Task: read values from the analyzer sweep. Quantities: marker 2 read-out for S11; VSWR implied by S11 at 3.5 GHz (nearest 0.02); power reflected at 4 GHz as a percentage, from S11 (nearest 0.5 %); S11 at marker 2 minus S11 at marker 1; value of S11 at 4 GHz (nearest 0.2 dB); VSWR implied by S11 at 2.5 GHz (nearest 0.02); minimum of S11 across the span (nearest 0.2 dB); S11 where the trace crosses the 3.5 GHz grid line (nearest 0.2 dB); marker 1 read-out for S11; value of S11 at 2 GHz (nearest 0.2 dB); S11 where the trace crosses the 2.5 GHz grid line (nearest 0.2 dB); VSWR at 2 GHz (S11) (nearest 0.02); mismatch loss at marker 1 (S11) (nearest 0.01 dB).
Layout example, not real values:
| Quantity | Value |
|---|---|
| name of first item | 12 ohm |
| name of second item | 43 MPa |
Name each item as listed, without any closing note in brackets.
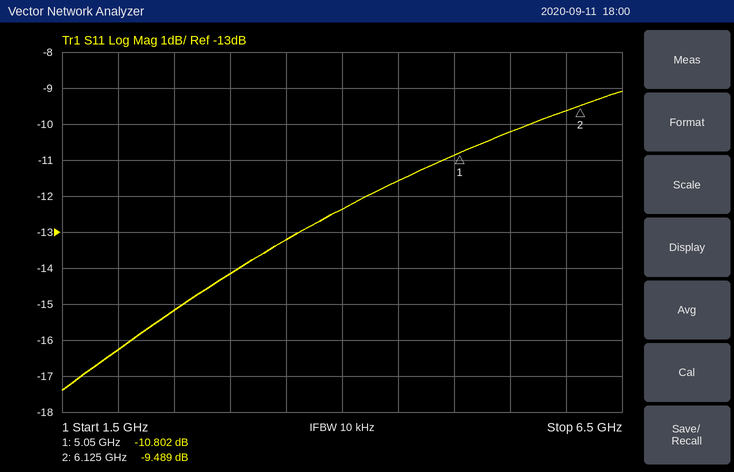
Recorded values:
| Quantity | Value |
|---|---|
| marker 2 read-out for S11 | -9.489 dB |
| VSWR implied by S11 at 3.5 GHz | 1.56 |
| power reflected at 4 GHz as a percentage, from S11 | 6.0 % |
| S11 at marker 2 minus S11 at marker 1 | 1.313 dB |
| value of S11 at 4 GHz | -12.4 dB |
| VSWR implied by S11 at 2.5 GHz | 1.42 |
| minimum of S11 across the span | -17.4 dB |
| S11 where the trace crosses the 3.5 GHz grid line | -13.2 dB |
| marker 1 read-out for S11 | -10.802 dB |
| value of S11 at 2 GHz | -16.2 dB |
| S11 where the trace crosses the 2.5 GHz grid line | -15.2 dB |
| VSWR at 2 GHz (S11) | 1.36 |
| mismatch loss at marker 1 (S11) | 0.38 dB |
